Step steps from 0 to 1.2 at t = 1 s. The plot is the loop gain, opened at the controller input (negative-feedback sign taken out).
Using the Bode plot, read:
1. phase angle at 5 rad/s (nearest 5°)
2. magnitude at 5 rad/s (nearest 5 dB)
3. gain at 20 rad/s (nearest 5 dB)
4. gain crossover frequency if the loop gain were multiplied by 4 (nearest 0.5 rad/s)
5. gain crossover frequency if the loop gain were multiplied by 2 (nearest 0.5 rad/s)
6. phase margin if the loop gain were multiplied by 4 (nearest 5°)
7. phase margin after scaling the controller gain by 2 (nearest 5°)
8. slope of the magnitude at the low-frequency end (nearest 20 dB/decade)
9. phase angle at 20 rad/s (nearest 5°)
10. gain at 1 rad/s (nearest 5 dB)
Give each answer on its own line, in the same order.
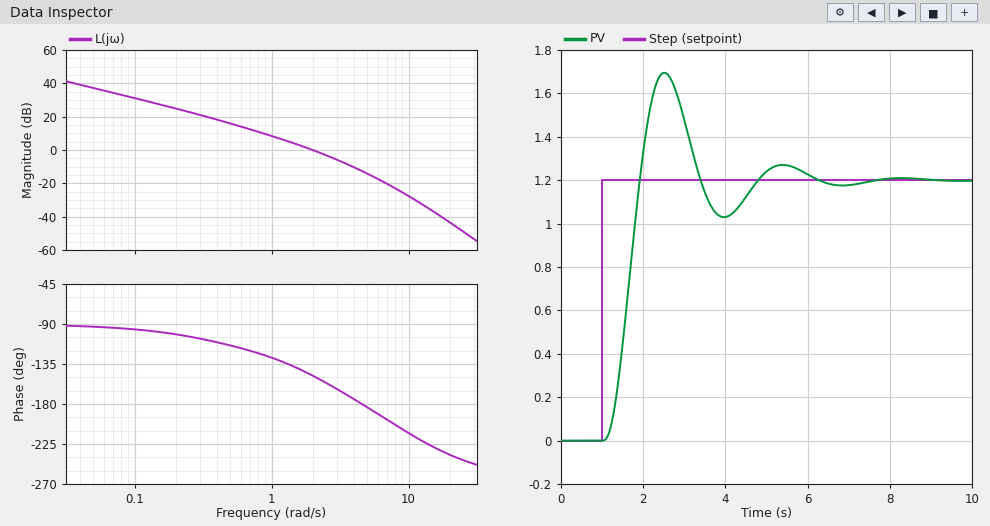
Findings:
-185°
-15 dB
-45 dB
4.5 rad/s
3.0 rad/s
0°
15°
-20 dB/decade
-235°
10 dB
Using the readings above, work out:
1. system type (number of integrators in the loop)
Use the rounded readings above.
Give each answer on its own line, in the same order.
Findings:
1
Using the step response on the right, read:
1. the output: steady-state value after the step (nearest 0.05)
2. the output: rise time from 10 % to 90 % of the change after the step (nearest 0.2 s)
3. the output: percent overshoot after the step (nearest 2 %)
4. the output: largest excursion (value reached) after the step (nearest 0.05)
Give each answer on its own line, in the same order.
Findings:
1.20
0.6 s
42 %
1.70
